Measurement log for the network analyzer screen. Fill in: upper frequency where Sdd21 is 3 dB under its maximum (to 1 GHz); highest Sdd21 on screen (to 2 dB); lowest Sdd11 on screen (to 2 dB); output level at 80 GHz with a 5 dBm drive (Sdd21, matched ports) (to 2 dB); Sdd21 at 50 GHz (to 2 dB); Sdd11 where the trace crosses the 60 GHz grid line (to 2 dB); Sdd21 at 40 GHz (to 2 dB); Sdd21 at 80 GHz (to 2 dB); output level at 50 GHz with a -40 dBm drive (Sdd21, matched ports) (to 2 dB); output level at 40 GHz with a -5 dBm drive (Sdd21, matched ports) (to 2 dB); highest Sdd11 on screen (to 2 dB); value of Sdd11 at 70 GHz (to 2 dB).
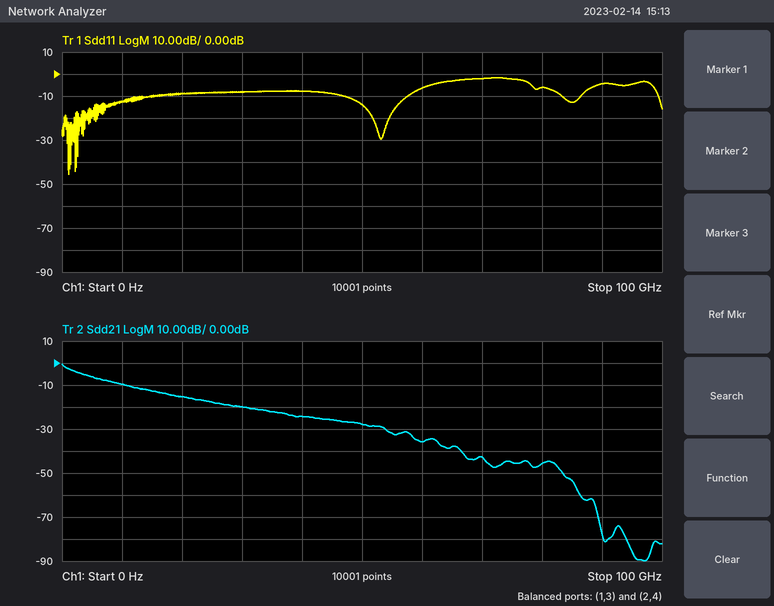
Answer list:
2 GHz
0 dB
-46 dB
-40 dBm
-28 dB
-6 dB
-24 dB
-46 dB
-68 dBm
-30 dBm
-2 dB
-2 dB
